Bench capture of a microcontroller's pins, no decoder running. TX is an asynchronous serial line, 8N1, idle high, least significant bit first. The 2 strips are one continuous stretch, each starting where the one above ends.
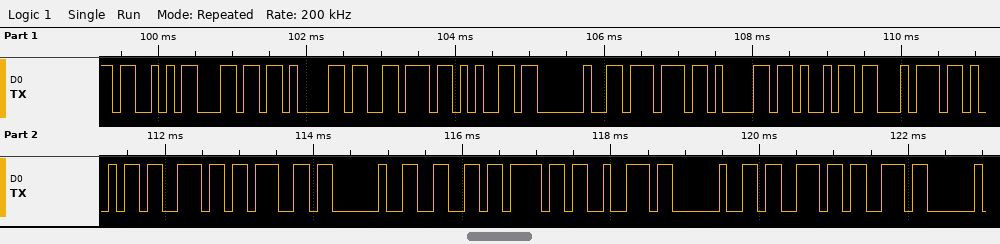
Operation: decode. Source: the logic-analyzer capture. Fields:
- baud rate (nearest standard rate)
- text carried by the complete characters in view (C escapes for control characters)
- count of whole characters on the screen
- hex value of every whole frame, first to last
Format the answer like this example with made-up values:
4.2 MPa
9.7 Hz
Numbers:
9600 baud
"Slave waiting for ss"
20
53 6C 61 76 65 20 77 61 69 74 69 6E 67 20 66 6F 72 20 73 73
